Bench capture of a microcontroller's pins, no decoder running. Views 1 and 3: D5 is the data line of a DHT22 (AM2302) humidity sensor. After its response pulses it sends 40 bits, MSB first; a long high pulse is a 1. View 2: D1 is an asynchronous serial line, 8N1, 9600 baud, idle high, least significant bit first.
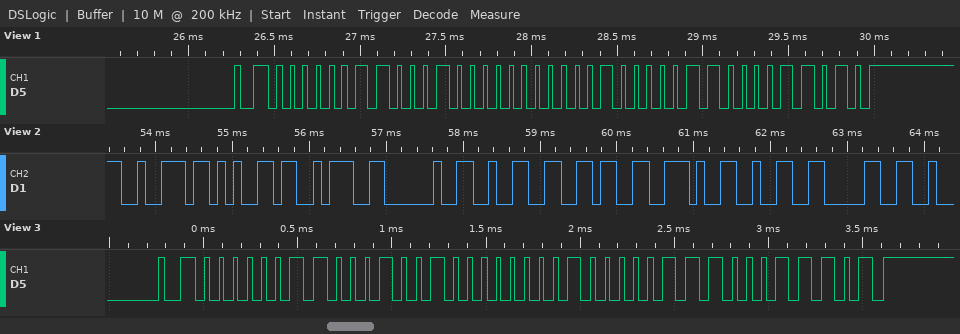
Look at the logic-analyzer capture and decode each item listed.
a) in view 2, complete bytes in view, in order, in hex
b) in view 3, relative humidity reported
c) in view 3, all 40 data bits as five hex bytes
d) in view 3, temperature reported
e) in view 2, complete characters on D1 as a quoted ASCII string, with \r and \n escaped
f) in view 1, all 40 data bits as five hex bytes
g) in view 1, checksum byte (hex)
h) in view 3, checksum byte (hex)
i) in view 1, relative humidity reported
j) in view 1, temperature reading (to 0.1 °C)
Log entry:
72 65 3A 20 32 36 2E 32 30
78.6 %
03 12 01 07 1D
26.3 °C
"re: 26.20"
03 10 01 06 1A
0x1A
0x1D
78.4 %
26.2 °C
